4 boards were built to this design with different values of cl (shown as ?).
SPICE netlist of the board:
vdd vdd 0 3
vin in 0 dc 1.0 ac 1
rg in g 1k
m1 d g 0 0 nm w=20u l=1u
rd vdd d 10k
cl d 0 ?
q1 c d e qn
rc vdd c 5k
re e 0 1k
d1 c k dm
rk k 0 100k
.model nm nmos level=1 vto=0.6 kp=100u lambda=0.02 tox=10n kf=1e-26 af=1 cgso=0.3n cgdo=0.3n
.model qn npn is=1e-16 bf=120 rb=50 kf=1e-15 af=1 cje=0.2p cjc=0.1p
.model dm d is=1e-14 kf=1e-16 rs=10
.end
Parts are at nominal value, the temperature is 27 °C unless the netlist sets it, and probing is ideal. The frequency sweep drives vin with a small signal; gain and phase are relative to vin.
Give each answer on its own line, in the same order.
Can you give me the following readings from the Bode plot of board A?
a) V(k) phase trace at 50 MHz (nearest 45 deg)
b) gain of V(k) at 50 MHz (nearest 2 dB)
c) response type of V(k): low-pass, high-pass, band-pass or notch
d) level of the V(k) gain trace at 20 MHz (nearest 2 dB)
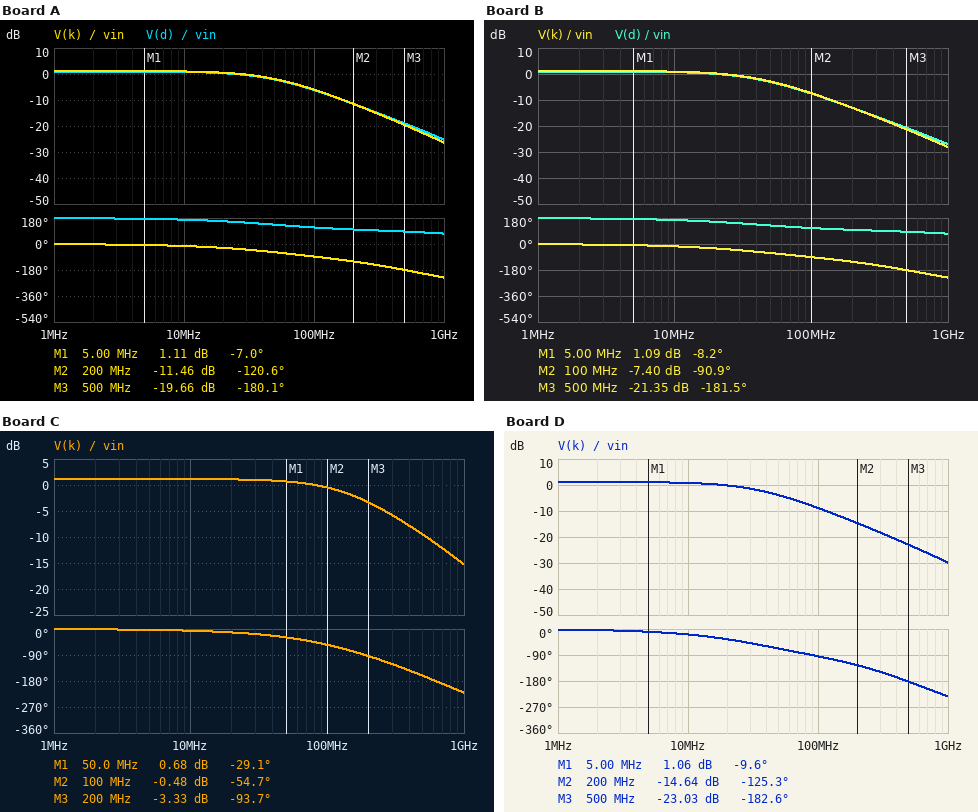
-45 deg
-2 dB
low-pass
0 dB
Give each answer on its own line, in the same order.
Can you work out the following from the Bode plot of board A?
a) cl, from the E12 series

2.2 pF
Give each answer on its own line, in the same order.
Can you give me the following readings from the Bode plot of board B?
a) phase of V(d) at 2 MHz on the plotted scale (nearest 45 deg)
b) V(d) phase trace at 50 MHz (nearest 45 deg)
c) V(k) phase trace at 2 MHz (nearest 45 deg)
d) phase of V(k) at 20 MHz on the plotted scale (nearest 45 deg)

180 deg
135 deg
0 deg
-45 deg
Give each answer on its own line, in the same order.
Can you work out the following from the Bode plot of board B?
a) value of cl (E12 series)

2.7 pF
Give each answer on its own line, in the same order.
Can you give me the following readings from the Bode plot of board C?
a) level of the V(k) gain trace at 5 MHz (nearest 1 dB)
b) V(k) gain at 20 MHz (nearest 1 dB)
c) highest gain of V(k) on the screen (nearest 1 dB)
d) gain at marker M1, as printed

1 dB
1 dB
1 dB
0.68 dB
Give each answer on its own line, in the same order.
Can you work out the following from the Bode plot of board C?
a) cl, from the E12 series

560 fF
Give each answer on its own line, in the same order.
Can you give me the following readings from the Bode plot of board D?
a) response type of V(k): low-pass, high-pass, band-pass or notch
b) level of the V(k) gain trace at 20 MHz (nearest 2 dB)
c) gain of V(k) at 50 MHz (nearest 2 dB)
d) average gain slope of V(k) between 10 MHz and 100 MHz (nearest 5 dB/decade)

low-pass
0 dB
-4 dB
-10 dB/decade
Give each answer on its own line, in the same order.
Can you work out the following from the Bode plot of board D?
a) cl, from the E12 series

3.3 pF
